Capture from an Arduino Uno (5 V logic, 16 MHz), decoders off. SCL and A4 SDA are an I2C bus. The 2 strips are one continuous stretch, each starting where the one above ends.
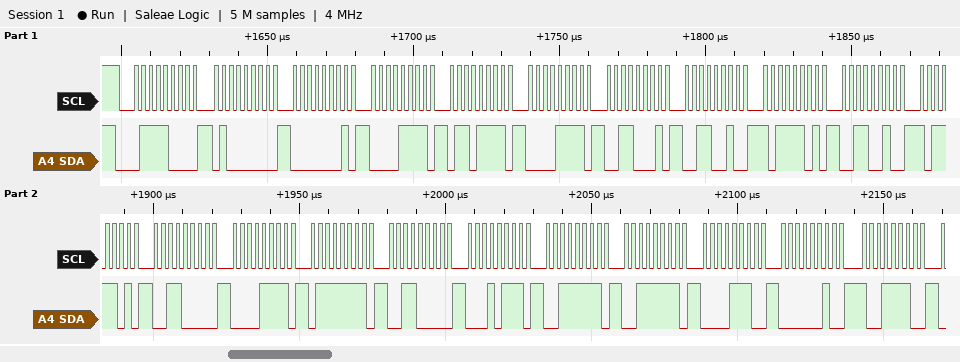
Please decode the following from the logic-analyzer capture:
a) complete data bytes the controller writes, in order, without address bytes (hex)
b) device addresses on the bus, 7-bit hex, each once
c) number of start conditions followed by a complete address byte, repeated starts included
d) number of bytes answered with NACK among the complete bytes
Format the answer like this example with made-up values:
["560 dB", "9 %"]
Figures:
["40 01 0F 6F 0F 31 32 BD 32 BD 30 0F 7F 30 17 3F 3F 0E 02 9E", "0x3C", "1", "0"]
